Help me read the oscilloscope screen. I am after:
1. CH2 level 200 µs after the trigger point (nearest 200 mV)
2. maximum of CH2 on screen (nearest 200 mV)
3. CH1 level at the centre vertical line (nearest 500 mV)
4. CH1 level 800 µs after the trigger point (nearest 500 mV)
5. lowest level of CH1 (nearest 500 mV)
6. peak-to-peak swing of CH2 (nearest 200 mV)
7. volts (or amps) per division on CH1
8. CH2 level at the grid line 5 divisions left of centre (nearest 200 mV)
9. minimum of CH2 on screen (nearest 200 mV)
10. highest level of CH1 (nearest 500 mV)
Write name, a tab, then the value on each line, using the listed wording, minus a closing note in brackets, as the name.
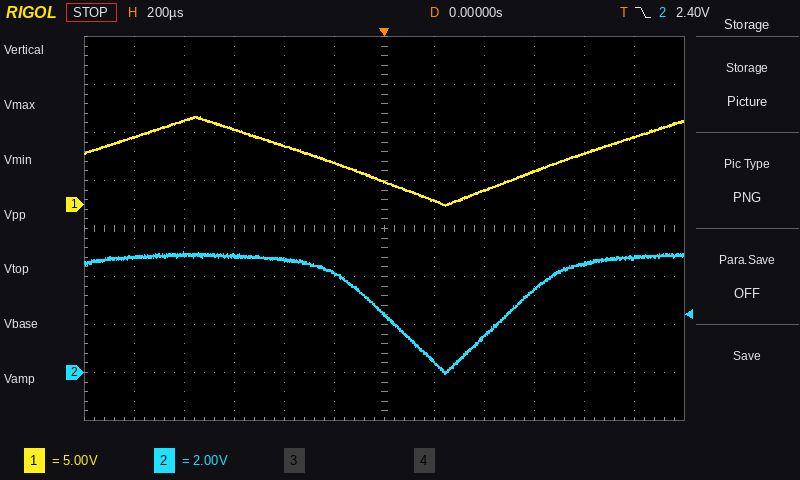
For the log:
CH2 level 200 µs after the trigger point	400 mV
maximum of CH2 on screen	5.0 V
CH1 level at the centre vertical line	2.5 V
CH1 level 800 µs after the trigger point	5.5 V
lowest level of CH1	0.0 V
peak-to-peak swing of CH2	5.0 V
volts (or amps) per division on CH1	5 V
CH2 level at the grid line 5 divisions left of centre	4.8 V
minimum of CH2 on screen	0.0 V
highest level of CH1	9.0 V
